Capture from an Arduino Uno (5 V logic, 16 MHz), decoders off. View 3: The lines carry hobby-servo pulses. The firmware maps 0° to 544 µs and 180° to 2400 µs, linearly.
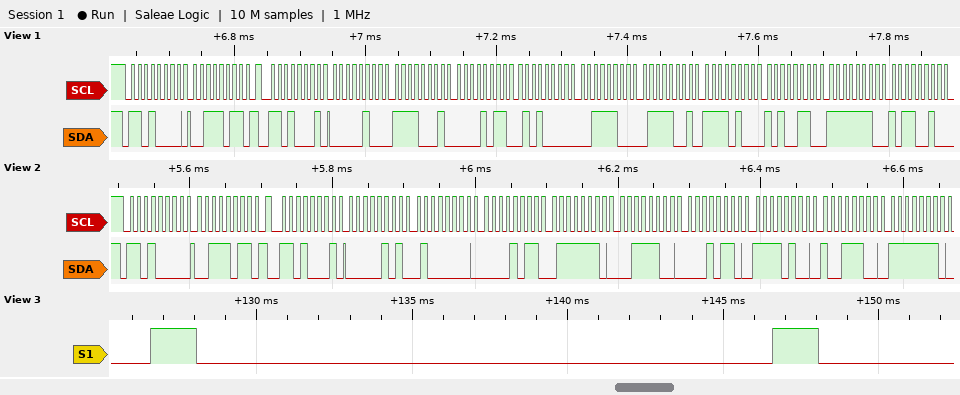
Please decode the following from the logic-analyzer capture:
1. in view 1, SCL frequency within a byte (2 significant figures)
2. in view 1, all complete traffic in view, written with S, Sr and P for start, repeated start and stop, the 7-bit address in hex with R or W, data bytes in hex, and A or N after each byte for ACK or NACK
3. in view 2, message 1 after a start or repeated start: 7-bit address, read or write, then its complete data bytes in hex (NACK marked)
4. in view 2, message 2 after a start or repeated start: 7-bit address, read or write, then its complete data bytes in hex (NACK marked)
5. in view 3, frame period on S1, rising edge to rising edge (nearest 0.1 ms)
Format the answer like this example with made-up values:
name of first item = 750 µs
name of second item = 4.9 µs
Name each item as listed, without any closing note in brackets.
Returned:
in view 1, SCL frequency within a byte = 100 kHz
in view 1, all complete traffic in view, written with S, Sr and P for start, repeated start and stop, the 7-bit address in hex with R or W, data bytes in hex, and A or N after each byte for ACK or NACK = S 68W A 3B A Sr 68R A 04 A F1 A 0B A 50 A 3C A 79 A F4 A A6 A FE A B2 A
in view 2, message 1 after a start or repeated start: 7-bit address, read or write, then its complete data bytes in hex = 0x68 write: 3B
in view 2, message 2 after a start or repeated start: 7-bit address, read or write, then its complete data bytes in hex = 0x68 read: 05 40 0B 7E 3C 16 F4 9C FE
in view 3, frame period on S1, rising edge to rising edge = 20.0 ms
